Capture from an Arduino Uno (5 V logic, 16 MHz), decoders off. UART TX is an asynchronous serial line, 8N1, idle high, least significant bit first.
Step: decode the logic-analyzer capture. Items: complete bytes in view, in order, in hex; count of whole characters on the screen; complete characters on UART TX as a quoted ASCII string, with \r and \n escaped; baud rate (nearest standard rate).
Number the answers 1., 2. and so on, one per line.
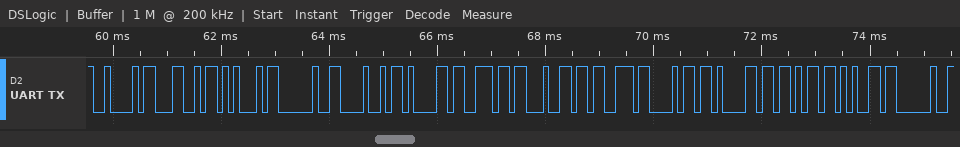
1. 0x42 0x4C 0x45 0x20 0x48 0x61 0x6E 0x64 0x73 0x68 0x61 0x6B 0x65 0x20
2. 14
3. "BLE Handshake "
4. 9600 baud
